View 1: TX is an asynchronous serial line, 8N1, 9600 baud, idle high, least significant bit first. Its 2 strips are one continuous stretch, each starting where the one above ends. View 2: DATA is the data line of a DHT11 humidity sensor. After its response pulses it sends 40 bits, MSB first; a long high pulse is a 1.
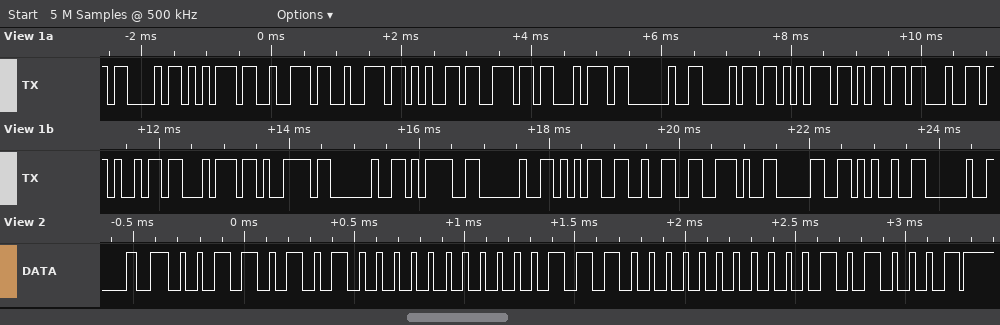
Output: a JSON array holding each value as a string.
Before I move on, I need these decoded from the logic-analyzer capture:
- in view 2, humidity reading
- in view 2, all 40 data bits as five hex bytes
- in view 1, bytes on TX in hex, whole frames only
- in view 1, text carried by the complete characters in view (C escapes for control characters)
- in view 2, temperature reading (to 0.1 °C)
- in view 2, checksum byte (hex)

["53 %", "35 00 1C 00 51", "43 75 72 72 65 6E 74 20 68 75 6D 64 69 74 79 20 3D 20 35 32 2E 30 25 20", "\"Current humdity = 52.0% \"", "28.0 °C", "0x51"]
